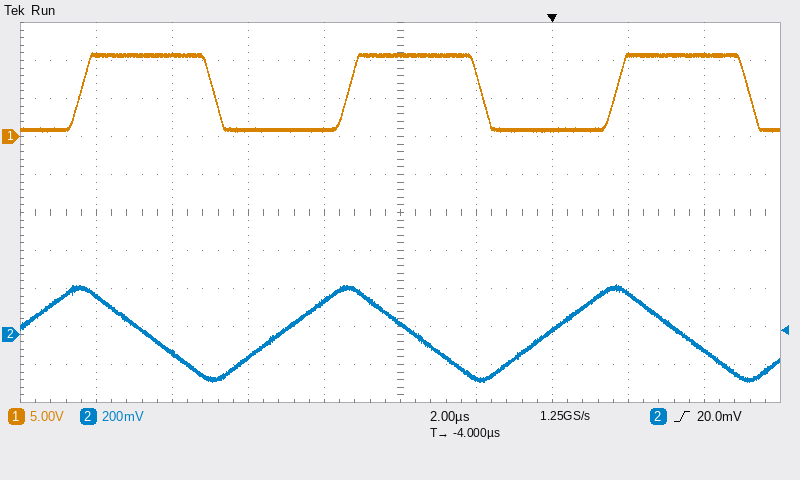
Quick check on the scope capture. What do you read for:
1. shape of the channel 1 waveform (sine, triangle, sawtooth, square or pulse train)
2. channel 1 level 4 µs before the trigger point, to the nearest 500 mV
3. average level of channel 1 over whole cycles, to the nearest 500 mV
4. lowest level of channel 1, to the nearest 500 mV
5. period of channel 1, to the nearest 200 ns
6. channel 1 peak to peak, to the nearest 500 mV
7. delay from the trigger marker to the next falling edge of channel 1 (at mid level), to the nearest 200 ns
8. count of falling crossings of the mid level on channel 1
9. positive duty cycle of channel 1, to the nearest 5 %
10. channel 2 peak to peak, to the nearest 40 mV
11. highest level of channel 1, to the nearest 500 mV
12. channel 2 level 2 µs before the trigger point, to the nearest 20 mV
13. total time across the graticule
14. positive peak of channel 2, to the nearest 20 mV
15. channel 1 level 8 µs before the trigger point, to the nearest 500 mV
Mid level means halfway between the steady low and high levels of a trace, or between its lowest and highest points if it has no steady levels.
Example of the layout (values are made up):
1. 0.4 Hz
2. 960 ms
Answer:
1. square
2. 10.5 V
3. 6.0 V
4. 500 mV
5. 7.0 µs
6. 10.5 V
7. 5.2 µs
8. 3
9. 50 %
10. 520 mV
11. 11.0 V
12. -240 mV
13. 20 µs
14. 260 mV
15. 1.0 V
